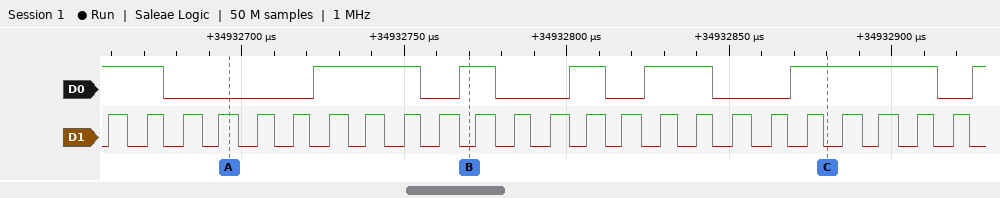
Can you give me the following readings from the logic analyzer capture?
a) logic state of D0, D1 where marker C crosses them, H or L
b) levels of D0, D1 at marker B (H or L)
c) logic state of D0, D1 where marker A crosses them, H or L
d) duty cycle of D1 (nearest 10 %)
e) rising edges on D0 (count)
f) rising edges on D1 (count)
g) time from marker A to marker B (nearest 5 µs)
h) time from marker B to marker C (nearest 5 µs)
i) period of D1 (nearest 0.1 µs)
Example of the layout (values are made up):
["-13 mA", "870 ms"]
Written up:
["D0=H, D1=L", "D0=H, D1=L", "D0=L, D1=H", "50 %", "6", "24", "75 µs", "110 µs", "11.3 µs"]
